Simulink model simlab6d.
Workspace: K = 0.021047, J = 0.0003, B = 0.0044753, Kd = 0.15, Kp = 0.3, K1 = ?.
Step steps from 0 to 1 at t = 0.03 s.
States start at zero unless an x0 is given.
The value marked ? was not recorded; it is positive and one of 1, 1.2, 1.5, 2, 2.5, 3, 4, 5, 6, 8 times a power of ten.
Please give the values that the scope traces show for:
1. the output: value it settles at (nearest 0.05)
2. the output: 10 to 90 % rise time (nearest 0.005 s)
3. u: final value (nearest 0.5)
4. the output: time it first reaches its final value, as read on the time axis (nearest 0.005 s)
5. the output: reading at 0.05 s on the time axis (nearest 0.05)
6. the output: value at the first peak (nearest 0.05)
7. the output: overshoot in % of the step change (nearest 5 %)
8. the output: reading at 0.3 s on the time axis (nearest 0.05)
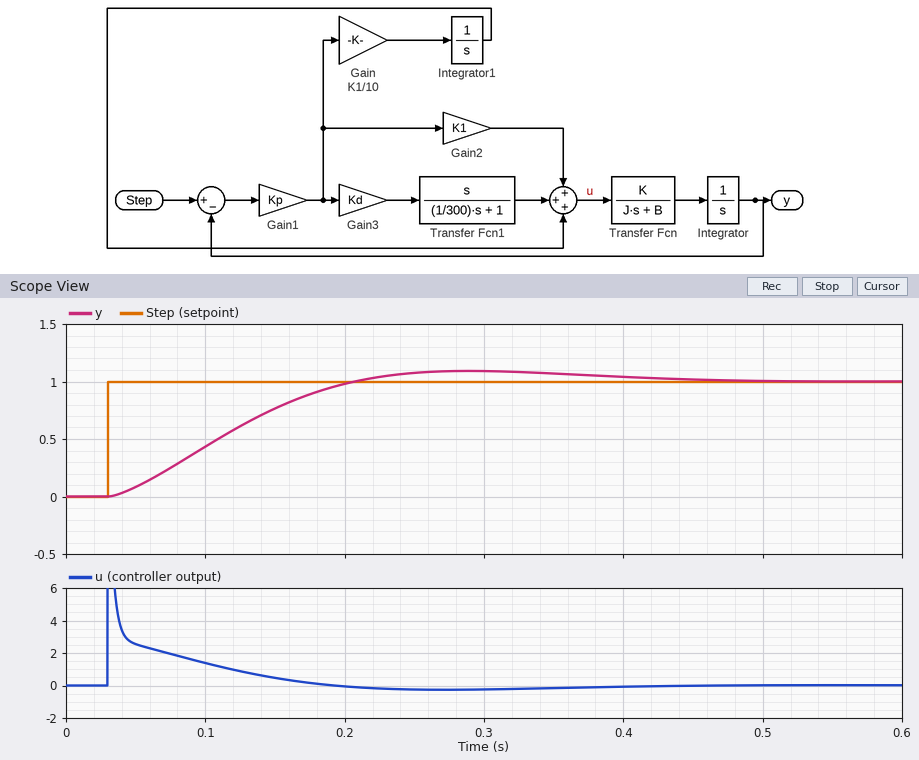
1.00
0.125 s
0.0
0.210 s
0.10
1.10
10 %
1.10
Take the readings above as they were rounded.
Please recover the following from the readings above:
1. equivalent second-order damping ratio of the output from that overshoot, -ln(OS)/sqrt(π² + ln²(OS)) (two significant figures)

0.59
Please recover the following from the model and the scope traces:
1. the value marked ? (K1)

10
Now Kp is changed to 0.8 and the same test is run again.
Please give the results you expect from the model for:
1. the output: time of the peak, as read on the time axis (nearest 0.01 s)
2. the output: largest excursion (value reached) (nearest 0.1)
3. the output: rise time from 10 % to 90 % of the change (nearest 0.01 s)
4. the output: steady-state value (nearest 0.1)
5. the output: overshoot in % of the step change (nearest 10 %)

0.16 s
1.2
0.06 s
1.0
20 %
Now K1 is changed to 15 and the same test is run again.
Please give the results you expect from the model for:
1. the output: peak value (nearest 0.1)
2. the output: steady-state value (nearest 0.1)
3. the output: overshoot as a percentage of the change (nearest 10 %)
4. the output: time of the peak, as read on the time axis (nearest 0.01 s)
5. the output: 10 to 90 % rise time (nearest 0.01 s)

1.2
1.0
20 %
0.22 s
0.09 s
